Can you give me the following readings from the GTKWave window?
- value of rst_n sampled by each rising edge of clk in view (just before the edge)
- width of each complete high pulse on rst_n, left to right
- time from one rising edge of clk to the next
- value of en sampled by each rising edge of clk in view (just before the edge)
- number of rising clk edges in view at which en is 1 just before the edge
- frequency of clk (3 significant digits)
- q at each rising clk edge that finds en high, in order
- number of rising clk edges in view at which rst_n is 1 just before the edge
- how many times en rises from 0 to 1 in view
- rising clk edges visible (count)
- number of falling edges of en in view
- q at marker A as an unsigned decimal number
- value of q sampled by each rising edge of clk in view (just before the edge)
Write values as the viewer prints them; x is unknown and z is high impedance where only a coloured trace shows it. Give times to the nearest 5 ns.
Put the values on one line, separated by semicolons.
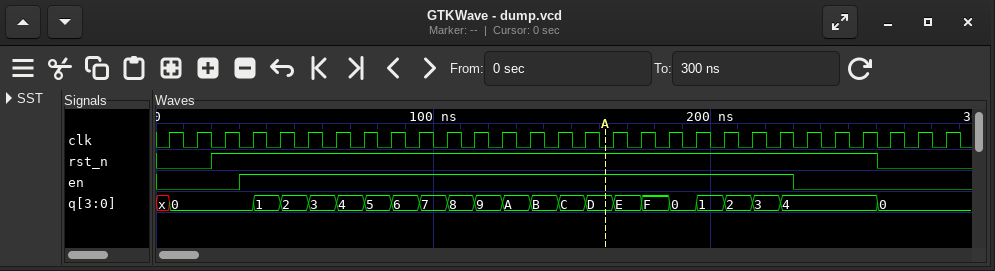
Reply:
0 0 1 1 1 1 1 1 1 1 1 1 1 1 1 1 1 1 1 1 1 1 1 1 1 1 0 0 0; 240 ns; 10 ns; 0 0 0 1 1 1 1 1 1 1 1 1 1 1 1 1 1 1 1 1 1 1 1 0 0 0 0 0 0; 20; 100 MHz; 0, 1, 2, 3, 4, 5, 6, 7, 8, 9, A, B, C, D, E, F, 0, 1, 2, 3; 24; 1; 29; 1; 13; x, 0, 0, 0, 1, 2, 3, 4, 5, 6, 7, 8, 9, A, B, C, D, E, F, 0, 1, 2, 3, 4, 4, 4, 0, 0, 0
